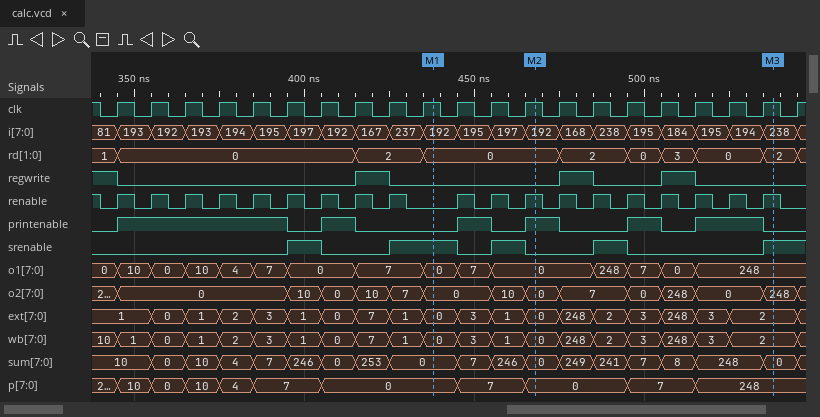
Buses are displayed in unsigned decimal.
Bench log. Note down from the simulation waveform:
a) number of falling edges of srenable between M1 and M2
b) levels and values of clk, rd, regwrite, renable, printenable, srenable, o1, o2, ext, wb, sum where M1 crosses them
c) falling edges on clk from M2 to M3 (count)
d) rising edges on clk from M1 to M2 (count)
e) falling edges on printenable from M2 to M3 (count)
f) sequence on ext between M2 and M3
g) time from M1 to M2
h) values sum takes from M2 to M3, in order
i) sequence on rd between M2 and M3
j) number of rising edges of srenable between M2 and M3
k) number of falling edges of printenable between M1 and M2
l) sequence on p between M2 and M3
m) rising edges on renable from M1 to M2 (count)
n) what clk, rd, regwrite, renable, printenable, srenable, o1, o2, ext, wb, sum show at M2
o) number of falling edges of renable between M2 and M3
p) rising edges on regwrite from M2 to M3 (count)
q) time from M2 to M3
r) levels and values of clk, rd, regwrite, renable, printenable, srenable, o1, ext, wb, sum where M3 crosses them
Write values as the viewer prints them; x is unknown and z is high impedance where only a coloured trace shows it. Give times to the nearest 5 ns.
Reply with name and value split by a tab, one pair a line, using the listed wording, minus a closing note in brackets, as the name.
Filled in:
number of falling edges of srenable between M1 and M2	2
levels and values of clk, rd, regwrite, renable, printenable, srenable, o1, o2, ext, wb, sum where M1 crosses them	clk=1, rd=0, regwrite=0, renable=0, printenable=0, srenable=1, o1=0, o2=0, ext=0, wb=0, sum=0
falling edges on clk from M2 to M3	7
rising edges on clk from M1 to M2	3
falling edges on printenable from M2 to M3	3
sequence on ext between M2 and M3	0, 248, 2, 3, 248, 3, 2
time from M1 to M2	30 ns
values sum takes from M2 to M3, in order	0, 249, 241, 7, 8, 248, 0
sequence on rd between M2 and M3	0, 2, 0, 3, 0, 2
number of rising edges of srenable between M2 and M3	2
number of falling edges of printenable between M1 and M2	1
sequence on p between M2 and M3	0, 7, 248
rising edges on renable from M1 to M2	3
what clk, rd, regwrite, renable, printenable, srenable, o1, o2, ext, wb, sum show at M2	clk=1, rd=0, regwrite=0, renable=1, printenable=1, srenable=0, o1=0, o2=0, ext=0, wb=0, sum=0
number of falling edges of renable between M2 and M3	7
rising edges on regwrite from M2 to M3	2
time from M2 to M3	70 ns
levels and values of clk, rd, regwrite, renable, printenable, srenable, o1, ext, wb, sum where M3 crosses them	clk=1, rd=2, regwrite=0, renable=1, printenable=0, srenable=1, o1=248, ext=2, wb=2, sum=0
